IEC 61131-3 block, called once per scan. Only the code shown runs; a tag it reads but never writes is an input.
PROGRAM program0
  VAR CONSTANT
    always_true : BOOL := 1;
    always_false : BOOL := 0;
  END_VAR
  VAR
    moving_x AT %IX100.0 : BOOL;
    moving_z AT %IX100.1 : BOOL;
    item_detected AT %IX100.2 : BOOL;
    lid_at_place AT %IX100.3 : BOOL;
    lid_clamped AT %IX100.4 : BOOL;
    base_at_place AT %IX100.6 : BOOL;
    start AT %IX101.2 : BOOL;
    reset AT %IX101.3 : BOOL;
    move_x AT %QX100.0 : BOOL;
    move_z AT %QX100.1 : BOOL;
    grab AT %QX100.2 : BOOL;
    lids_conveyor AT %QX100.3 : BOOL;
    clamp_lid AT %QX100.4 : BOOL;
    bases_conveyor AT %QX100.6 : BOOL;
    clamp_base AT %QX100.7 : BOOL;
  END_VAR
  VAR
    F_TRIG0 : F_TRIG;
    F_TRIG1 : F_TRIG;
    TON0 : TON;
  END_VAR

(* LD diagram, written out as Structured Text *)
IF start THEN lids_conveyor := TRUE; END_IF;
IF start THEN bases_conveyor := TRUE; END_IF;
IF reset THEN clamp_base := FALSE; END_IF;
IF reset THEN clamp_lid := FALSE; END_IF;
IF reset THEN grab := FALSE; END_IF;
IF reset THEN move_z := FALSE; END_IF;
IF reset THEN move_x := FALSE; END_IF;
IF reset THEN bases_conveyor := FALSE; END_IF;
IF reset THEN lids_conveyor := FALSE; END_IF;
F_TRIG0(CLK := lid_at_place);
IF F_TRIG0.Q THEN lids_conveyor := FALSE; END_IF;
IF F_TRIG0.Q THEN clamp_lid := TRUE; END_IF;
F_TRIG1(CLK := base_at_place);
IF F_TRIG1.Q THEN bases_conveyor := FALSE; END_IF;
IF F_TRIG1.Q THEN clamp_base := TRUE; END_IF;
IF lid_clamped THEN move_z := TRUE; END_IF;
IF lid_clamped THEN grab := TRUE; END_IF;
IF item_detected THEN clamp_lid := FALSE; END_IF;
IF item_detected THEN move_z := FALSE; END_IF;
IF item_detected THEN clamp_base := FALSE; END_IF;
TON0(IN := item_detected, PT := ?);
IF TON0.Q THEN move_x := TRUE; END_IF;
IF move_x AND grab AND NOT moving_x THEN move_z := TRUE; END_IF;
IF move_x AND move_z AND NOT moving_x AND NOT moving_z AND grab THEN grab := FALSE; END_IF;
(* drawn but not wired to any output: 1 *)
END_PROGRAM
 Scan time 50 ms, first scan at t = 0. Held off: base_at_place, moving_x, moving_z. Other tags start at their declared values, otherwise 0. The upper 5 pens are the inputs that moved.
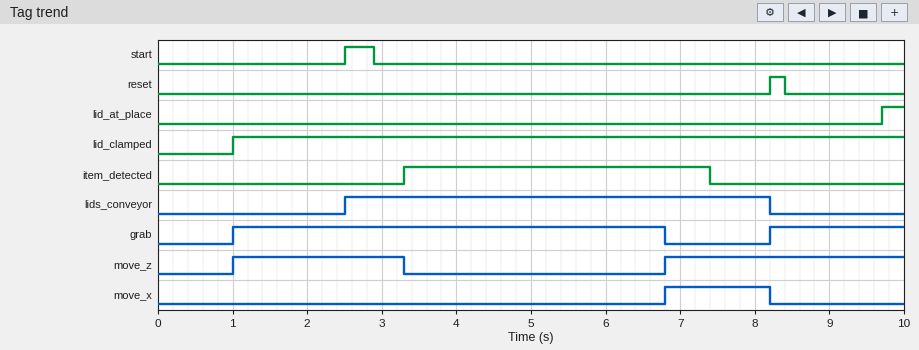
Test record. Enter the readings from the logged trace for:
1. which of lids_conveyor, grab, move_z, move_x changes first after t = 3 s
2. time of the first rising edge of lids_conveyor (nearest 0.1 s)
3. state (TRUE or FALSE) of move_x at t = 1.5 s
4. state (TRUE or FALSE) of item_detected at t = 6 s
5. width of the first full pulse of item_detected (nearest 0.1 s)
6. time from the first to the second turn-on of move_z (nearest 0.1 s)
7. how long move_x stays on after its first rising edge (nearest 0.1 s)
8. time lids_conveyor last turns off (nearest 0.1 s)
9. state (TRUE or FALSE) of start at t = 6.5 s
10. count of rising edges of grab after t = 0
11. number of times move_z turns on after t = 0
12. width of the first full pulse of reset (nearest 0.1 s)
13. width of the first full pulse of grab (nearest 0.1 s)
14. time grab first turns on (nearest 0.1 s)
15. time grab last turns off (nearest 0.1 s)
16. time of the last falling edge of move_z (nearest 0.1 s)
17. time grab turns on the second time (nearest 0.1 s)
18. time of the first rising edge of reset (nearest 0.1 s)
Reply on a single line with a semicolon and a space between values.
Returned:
move_z; 2.5 s; FALSE; TRUE; 4.1 s; 5.8 s; 1.4 s; 8.2 s; FALSE; 2; 2; 0.2 s; 5.8 s; 1.0 s; 6.8 s; 3.3 s; 8.2 s; 8.2 s
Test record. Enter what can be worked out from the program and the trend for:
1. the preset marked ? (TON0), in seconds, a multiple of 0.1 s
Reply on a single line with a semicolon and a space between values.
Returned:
3.5 s
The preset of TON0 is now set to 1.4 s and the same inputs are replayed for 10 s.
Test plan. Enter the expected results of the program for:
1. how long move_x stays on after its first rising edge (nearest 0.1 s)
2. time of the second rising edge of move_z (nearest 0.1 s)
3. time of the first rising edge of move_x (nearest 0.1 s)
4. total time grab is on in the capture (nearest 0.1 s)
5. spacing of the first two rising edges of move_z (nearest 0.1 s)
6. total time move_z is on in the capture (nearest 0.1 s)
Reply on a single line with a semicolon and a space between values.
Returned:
3.5 s; 4.7 s; 4.7 s; 5.5 s; 3.7 s; 7.6 s
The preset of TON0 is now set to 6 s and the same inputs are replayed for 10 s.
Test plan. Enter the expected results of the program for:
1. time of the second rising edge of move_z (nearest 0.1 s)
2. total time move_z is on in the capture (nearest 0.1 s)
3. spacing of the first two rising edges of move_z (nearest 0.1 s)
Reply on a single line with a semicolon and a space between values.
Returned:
7.4 s; 4.9 s; 6.4 s
